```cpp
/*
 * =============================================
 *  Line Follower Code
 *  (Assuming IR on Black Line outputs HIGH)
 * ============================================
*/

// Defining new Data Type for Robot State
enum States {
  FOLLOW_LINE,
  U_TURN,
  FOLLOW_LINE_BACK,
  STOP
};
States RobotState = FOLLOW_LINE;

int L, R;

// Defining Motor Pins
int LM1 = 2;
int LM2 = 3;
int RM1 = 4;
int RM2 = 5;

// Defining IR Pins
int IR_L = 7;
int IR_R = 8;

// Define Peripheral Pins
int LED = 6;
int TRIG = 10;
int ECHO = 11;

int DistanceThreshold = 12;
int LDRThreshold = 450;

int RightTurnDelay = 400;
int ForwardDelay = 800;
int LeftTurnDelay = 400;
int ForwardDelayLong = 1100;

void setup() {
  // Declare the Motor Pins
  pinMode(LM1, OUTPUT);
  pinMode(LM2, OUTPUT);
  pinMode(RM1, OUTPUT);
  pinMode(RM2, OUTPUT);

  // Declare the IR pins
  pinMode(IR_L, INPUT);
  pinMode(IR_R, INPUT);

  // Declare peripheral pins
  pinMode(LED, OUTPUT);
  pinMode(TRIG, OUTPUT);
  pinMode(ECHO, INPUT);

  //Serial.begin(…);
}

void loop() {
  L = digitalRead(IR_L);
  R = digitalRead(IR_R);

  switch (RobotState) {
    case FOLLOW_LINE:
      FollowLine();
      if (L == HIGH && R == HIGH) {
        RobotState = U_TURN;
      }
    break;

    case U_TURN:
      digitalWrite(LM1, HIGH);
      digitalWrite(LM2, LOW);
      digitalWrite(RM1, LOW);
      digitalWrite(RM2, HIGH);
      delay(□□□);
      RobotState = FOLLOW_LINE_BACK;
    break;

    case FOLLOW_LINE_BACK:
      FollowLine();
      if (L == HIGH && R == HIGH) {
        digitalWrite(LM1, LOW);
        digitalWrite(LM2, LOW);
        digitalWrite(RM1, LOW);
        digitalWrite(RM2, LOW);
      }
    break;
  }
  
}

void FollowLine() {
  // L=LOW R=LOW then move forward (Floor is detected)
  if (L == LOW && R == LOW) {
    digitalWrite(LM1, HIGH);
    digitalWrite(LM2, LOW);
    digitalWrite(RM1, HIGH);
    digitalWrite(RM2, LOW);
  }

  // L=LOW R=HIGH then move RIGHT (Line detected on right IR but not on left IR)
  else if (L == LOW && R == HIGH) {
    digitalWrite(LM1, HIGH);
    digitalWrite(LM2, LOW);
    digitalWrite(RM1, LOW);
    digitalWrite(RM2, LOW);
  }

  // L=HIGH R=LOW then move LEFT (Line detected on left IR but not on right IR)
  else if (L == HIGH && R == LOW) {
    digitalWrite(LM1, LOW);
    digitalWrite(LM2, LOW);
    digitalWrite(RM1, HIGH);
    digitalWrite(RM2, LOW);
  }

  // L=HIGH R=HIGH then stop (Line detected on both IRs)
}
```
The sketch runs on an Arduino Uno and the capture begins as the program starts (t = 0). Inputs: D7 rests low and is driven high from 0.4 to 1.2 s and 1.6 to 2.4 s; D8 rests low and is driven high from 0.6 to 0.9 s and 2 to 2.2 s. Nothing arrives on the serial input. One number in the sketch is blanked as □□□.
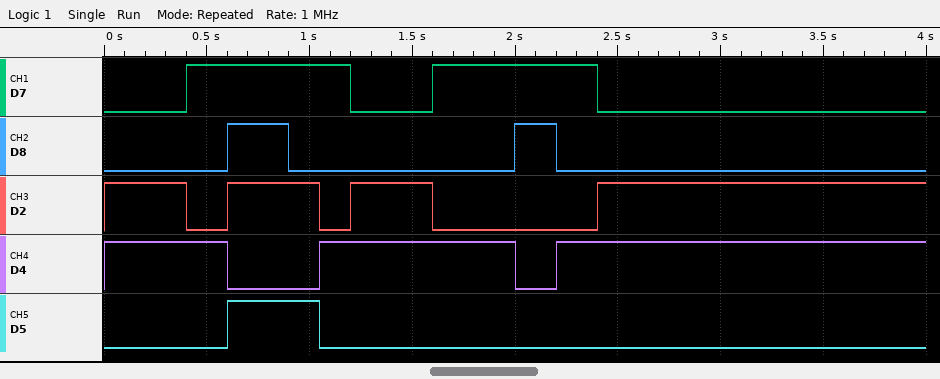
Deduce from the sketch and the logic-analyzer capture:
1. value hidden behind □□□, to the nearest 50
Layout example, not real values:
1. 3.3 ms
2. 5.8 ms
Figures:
1. 450
